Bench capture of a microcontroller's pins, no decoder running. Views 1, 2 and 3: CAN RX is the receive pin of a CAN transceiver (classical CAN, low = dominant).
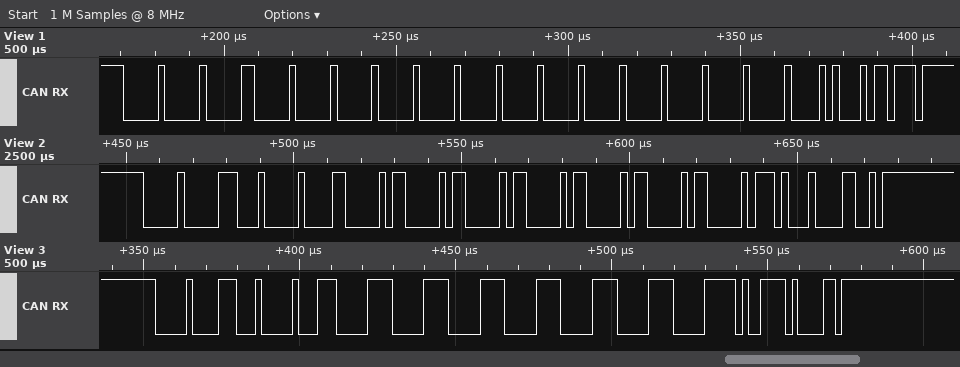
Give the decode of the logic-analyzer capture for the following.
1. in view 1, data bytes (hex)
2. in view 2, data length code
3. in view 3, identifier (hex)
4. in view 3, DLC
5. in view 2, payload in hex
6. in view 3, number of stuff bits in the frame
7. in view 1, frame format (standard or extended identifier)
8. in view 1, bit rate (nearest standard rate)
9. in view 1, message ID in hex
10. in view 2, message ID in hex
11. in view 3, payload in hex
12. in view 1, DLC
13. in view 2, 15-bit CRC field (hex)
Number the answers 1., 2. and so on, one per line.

1. 00 00 00 00 00 00 00 00
2. 8
3. 0x007
4. 8
5. 03 03 03 03 03 03 03 03
6. 10
7. standard
8. 500 kbit/s
9. 0x000
10. 0x003
11. 07 07 07 07 07 07 07 07
12. 8
13. 0x510C
